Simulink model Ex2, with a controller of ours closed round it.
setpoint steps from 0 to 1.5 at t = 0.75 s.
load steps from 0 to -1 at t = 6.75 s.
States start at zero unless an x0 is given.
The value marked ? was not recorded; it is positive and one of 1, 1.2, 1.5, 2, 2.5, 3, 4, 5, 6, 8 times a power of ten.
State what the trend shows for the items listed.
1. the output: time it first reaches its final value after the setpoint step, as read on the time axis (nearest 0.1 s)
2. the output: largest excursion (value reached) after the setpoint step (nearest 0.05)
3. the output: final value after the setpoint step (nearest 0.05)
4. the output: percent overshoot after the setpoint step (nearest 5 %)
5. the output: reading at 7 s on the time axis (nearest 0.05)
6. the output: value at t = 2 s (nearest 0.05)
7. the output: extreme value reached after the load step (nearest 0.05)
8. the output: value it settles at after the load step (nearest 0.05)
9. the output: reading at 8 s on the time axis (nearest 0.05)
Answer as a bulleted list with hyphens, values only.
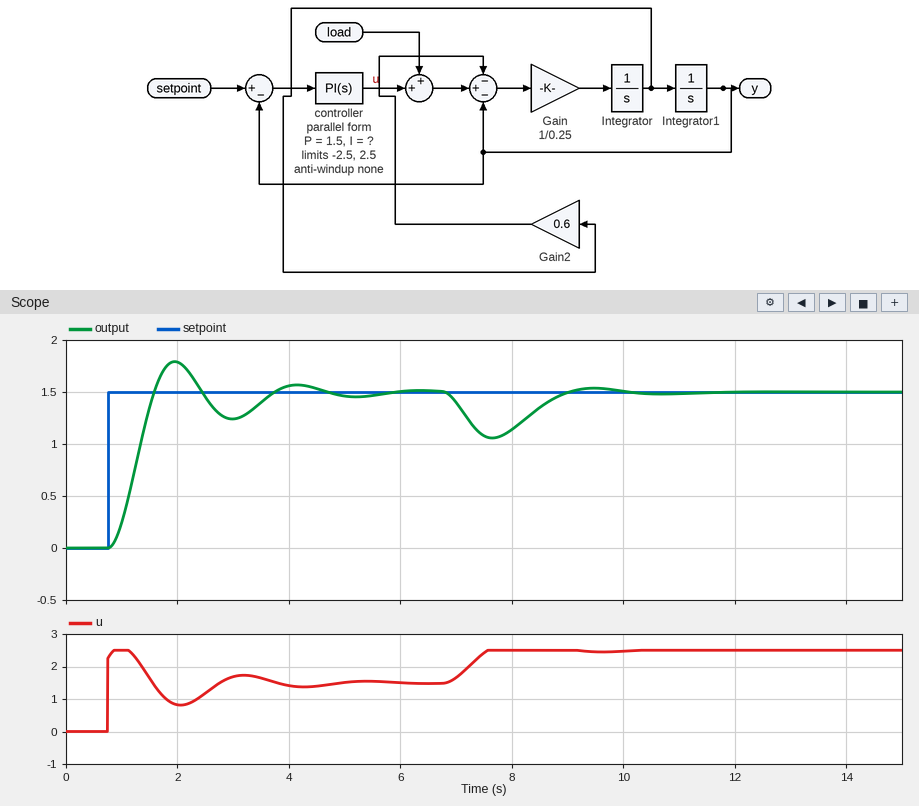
- 1.6 s
- 1.80
- 1.50
- 20 %
- 1.40
- 1.80
- 1.05
- 1.50
- 1.15
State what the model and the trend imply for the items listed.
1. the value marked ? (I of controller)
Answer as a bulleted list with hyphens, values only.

- 2
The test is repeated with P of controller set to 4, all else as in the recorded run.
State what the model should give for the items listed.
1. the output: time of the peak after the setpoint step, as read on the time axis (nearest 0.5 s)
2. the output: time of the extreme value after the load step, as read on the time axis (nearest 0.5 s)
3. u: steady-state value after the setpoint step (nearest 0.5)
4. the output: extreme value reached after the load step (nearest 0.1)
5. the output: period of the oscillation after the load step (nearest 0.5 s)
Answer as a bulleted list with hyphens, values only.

- 2.0 s
- 7.5 s
- 1.5
- 1.2
- 2.0 s
